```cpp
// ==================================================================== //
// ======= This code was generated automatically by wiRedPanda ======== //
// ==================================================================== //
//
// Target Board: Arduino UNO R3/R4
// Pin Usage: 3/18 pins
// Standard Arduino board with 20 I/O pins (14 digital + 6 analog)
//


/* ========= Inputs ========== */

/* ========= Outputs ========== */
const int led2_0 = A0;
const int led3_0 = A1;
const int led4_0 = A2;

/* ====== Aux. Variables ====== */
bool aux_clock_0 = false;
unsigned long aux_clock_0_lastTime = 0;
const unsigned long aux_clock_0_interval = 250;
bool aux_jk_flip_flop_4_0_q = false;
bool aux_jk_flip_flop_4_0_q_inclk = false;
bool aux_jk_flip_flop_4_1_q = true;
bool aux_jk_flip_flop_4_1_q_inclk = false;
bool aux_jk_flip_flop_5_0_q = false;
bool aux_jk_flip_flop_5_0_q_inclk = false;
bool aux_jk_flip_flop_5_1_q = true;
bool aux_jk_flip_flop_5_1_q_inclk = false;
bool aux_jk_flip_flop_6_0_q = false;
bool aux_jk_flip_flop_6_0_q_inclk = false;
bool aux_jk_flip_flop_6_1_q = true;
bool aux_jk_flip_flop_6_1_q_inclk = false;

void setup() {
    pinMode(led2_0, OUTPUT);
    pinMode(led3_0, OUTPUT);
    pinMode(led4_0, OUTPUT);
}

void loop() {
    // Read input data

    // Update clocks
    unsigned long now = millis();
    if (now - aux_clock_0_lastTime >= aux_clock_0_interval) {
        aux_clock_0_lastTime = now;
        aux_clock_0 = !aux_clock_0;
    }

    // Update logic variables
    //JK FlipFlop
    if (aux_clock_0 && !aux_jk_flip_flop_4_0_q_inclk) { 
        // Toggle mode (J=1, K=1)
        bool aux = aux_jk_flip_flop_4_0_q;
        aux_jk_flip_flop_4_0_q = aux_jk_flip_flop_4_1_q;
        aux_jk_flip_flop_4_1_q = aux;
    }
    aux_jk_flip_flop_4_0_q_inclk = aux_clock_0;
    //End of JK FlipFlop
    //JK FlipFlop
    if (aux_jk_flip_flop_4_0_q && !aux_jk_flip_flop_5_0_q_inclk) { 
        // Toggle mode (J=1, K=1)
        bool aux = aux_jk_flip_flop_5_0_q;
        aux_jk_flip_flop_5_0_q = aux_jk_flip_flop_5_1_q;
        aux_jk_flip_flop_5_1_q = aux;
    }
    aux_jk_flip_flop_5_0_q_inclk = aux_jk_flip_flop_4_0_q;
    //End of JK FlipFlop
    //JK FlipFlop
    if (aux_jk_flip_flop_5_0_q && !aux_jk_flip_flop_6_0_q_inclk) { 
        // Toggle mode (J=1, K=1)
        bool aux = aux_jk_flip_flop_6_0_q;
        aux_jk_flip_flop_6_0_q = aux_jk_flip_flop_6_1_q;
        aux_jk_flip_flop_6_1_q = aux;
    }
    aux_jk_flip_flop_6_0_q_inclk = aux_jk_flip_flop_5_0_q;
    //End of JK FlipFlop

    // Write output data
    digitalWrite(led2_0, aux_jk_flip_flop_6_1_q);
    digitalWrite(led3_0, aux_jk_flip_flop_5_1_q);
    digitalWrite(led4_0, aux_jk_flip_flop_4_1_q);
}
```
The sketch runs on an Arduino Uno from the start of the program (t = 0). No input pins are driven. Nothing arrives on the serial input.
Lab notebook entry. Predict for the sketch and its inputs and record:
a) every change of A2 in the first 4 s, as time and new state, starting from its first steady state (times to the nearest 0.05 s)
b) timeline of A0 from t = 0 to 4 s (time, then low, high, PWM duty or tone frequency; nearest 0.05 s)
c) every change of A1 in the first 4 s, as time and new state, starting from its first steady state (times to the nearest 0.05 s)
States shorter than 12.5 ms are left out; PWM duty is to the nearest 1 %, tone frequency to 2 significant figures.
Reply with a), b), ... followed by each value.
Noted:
a) 0 s high; 0.25 s low; 0.75 s high; 1.25 s low; 1.75 s high; 2.25 s low; 2.75 s high; 3.25 s low; 3.75 s high
b) 0 s high; 0.25 s low; 2.25 s high
c) 0 s high; 0.25 s low; 1.25 s high; 2.25 s low; 3.25 s high
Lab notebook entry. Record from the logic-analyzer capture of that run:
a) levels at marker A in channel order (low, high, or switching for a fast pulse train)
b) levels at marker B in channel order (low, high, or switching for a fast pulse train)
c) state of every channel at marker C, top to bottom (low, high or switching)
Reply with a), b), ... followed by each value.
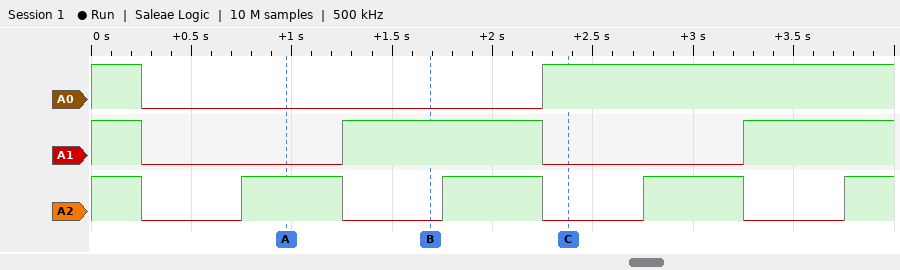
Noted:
a) A0 low, A1 low, A2 high
b) A0 low, A1 high, A2 low
c) A0 high, A1 low, A2 low
